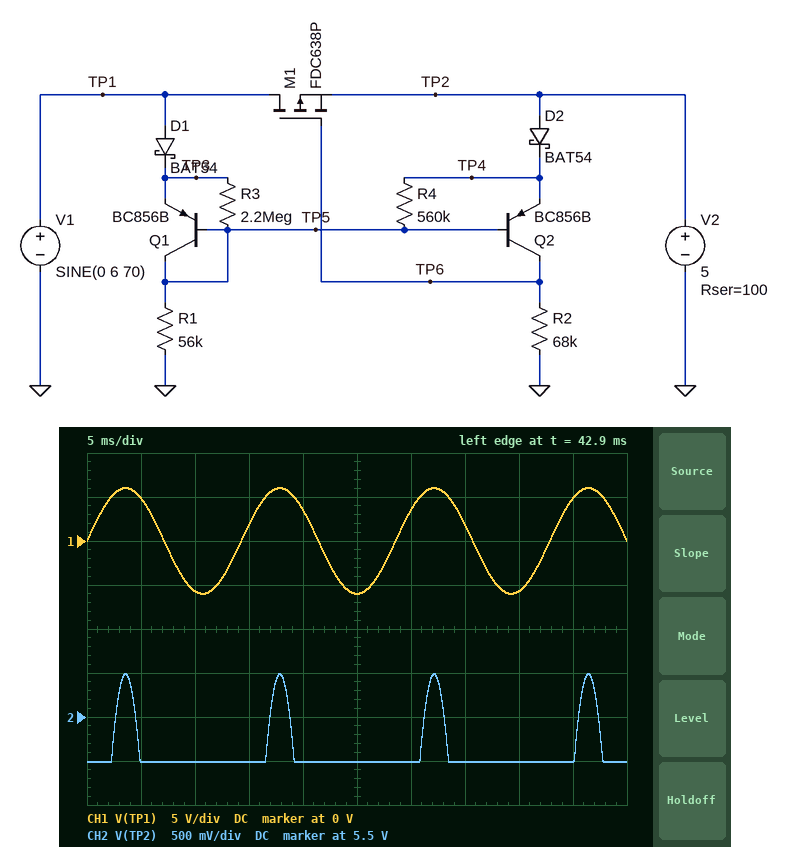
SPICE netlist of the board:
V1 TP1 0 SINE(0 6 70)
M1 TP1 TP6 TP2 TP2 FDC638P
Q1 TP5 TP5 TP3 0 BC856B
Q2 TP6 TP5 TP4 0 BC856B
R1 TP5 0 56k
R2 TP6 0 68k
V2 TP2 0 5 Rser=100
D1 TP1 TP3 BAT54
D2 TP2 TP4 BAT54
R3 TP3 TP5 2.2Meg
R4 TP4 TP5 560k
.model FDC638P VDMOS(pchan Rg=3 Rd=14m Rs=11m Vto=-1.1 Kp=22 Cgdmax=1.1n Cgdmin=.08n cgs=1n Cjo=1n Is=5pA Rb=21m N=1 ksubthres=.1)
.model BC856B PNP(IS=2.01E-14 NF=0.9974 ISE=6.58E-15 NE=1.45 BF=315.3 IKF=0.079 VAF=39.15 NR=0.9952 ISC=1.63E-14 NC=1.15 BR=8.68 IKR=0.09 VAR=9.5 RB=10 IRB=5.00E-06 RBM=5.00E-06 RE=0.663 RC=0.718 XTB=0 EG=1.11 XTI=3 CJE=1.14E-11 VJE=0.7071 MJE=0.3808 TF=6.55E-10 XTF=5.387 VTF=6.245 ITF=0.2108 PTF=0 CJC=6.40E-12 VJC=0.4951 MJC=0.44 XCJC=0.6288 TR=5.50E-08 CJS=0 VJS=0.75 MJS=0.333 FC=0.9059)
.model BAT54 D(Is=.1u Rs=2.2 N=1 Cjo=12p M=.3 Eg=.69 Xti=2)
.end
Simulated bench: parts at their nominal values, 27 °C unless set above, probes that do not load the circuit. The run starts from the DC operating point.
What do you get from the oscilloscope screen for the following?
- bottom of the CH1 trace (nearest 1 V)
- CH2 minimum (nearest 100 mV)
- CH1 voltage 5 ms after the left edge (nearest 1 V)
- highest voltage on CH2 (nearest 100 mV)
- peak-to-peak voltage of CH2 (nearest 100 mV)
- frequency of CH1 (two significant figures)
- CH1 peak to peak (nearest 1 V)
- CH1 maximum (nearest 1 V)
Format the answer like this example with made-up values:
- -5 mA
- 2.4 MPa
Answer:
- -6 V
- 5.0 V
- 5 V
- 6.0 V
- 1.0 V
- 70 Hz
- 12 V
- 6 V
